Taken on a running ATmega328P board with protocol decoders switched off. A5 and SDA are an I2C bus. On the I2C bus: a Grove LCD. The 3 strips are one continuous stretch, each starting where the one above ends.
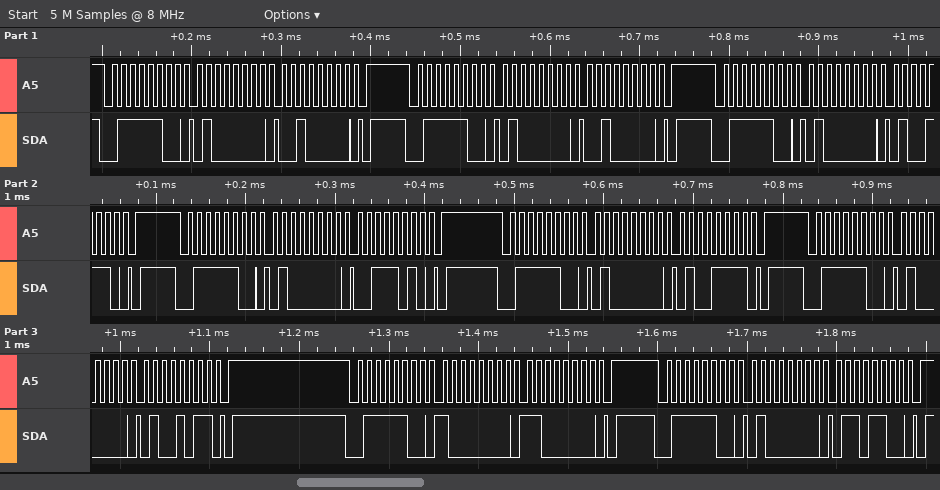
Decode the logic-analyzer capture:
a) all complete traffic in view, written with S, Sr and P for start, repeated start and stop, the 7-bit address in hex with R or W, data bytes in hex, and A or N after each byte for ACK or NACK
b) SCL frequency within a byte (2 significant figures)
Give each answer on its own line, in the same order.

S 3EW A 40 A 20 A P S 3EW A 40 A 20 A P S 3EW A 40 A 4E A P S 3EW A 40 A 3A A P S 3EW A 40 A 4F A P S 3EW A 40 A 4B A P S 3EW A 80 A C0 A P S 3EW A 40 A 6C A P
100 kHz
